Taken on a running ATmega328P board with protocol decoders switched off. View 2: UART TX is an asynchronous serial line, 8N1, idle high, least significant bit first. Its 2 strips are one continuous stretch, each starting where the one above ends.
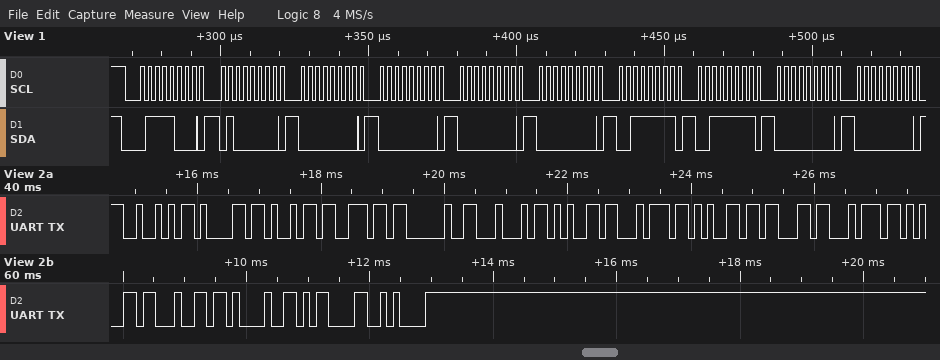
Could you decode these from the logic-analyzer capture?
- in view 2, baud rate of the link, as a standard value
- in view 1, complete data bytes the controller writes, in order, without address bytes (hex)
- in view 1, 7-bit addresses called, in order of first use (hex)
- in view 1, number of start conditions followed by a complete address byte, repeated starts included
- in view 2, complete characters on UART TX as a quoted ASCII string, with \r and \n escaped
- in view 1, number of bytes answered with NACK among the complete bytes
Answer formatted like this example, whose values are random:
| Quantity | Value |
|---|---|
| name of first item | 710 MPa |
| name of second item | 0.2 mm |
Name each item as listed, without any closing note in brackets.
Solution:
| Quantity | Value |
|---|---|
| in view 2, baud rate of the link, as a standard value | 9600 baud |
| in view 1, complete data bytes the controller writes, in order, without address bytes | 40 00 00 00 00 3F 3F 00 00 |
| in view 1, 7-bit addresses called, in order of first use | 0x3C |
| in view 1, number of start conditions followed by a complete address byte, repeated starts included | 1 |
| in view 2, complete characters on UART TX as a quoted ASCII string, with \r and \n escaped | "Rain Detected!\r\n" |
| in view 1, number of bytes answered with NACK among the complete bytes | 0 |
